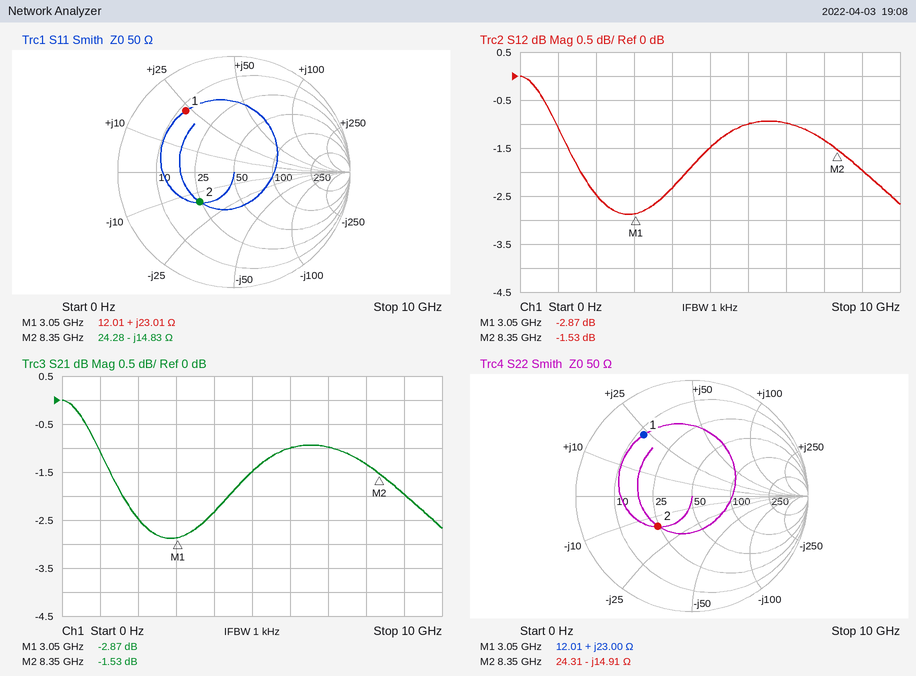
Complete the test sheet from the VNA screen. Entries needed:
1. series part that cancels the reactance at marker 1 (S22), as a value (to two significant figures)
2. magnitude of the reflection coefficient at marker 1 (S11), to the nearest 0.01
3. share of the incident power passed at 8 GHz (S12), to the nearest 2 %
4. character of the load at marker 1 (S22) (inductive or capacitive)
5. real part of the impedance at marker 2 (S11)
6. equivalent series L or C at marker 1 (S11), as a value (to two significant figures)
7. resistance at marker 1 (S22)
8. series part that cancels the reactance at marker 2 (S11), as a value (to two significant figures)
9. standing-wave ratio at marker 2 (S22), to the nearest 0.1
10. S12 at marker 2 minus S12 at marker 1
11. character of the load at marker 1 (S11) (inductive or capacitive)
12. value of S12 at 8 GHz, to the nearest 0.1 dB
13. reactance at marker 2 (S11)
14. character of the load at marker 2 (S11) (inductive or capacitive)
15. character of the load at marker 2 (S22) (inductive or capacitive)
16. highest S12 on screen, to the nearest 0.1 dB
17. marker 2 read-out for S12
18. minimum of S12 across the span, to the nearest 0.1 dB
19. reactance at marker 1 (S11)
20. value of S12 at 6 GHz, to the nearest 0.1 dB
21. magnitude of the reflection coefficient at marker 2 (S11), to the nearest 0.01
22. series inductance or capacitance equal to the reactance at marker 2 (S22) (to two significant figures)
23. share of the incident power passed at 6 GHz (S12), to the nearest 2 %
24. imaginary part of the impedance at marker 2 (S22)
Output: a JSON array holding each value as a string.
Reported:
["2.3 pF", "0.67", "74 %", "inductive", "24.28 Ω", "1.2 nH", "12.01 Ω", "280 pH", "2.3", "1.34 dB", "inductive", "-1.3 dB", "-14.83 Ω", "capacitive", "capacitive", "0.0 dB", "-1.53 dB", "-2.9 dB", "+23.01 Ω", "-1.0 dB", "0.39", "1.3 pF", "80 %", "-14.91 Ω"]
